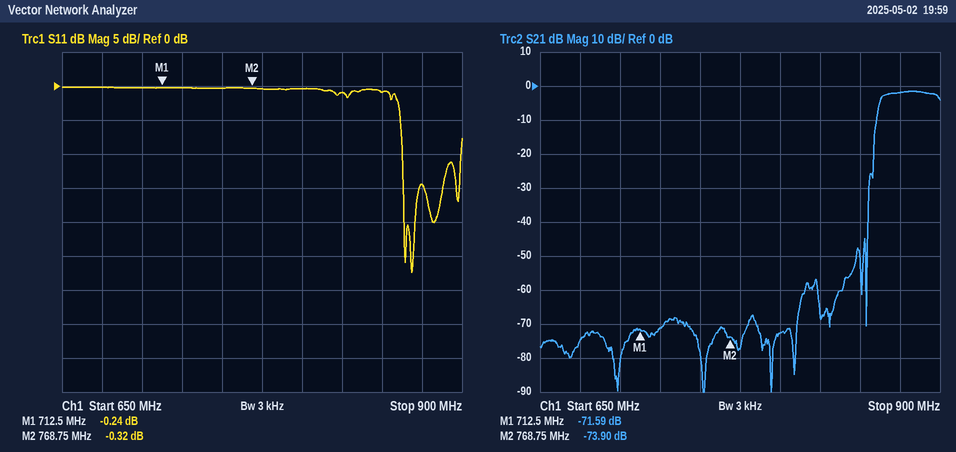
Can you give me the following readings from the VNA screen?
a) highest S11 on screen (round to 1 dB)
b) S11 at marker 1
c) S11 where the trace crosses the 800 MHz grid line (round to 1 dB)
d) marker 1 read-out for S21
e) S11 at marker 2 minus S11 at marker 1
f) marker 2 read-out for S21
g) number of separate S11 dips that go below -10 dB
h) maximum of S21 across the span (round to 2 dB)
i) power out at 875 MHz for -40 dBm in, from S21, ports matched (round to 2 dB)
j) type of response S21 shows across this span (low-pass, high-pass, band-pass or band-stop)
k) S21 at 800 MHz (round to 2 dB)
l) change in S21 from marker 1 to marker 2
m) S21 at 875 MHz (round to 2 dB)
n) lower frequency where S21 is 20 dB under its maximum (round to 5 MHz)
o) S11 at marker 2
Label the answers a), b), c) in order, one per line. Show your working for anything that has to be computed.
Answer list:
a) 0 dB
b) -0.24 dB
c) 0 dB
d) -71.59 dB
e) -0.32 − (-0.24) = -0.08 dB
f) -73.90 dB
g) 4
h) -2 dB
i) -40 dBm + (-2 dB) = -42 dBm
j) high-pass
k) -72 dB
l) -73.9 − (-71.59) = -2.31 dB
m) -2 dB
n) 860 MHz
o) -0.32 dB
